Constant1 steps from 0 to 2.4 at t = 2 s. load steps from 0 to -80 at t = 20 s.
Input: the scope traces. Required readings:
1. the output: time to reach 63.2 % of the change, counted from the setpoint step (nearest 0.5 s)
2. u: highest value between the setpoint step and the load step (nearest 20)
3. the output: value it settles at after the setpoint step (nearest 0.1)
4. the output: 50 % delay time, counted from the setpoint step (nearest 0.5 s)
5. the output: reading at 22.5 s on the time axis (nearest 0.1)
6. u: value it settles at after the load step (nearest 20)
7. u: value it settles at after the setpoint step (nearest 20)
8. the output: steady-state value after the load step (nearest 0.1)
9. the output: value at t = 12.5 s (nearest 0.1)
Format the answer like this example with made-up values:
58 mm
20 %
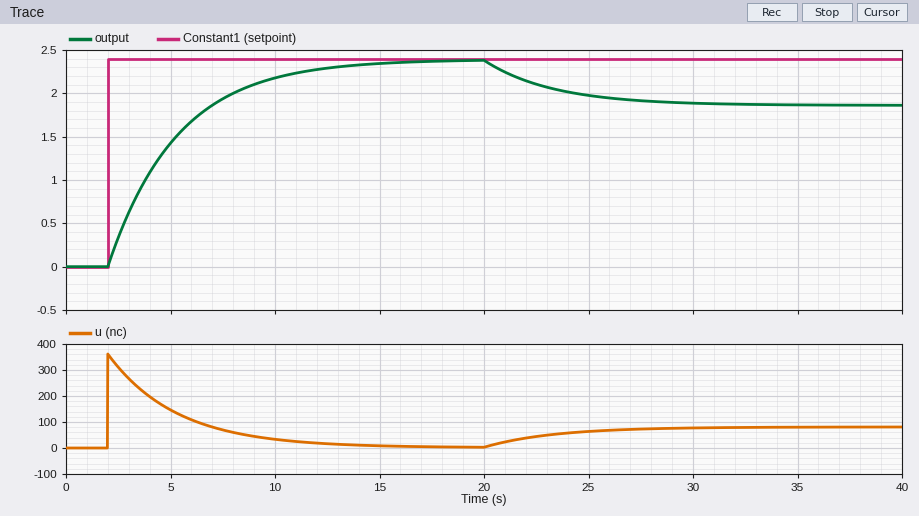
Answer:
3.5 s
360
2.4
2.5 s
2.1
80
0
1.9
2.3
